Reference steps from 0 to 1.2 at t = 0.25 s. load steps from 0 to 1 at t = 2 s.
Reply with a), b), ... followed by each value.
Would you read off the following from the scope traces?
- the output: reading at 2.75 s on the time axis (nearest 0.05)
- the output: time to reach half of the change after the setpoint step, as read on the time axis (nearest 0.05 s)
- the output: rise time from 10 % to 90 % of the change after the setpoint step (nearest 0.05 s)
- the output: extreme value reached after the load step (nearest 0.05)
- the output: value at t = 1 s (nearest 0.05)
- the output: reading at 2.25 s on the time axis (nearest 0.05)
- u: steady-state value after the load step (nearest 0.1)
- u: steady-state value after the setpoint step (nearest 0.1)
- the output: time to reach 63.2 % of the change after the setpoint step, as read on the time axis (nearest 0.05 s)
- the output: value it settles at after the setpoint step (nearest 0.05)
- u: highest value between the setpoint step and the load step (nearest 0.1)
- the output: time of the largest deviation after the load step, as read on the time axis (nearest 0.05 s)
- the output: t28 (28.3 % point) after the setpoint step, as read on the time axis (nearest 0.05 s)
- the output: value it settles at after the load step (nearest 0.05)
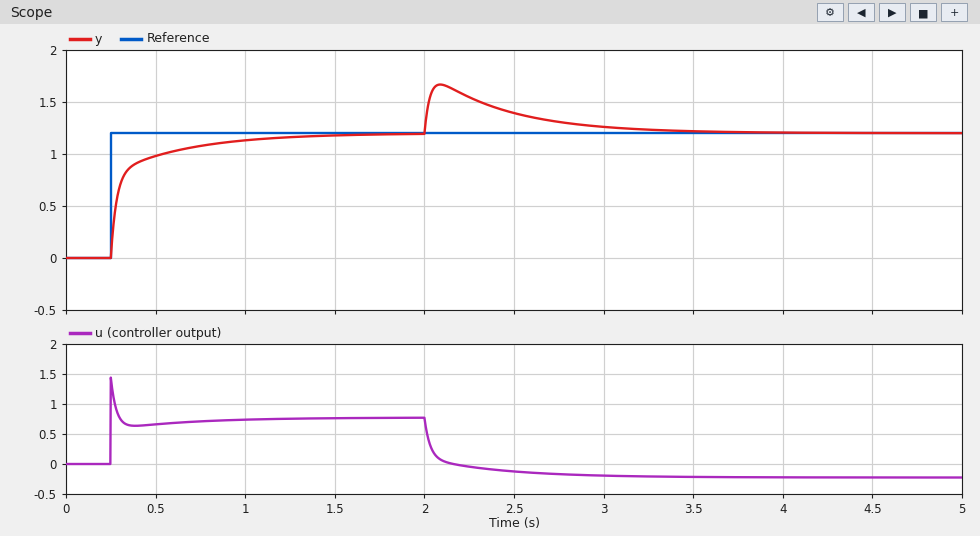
a) 1.30
b) 0.30 s
c) 0.50 s
d) 1.65
e) 1.15
f) 1.55
g) -0.2
h) 0.8
i) 0.30 s
j) 1.20
k) 1.4
l) 2.10 s
m) 0.25 s
n) 1.20
